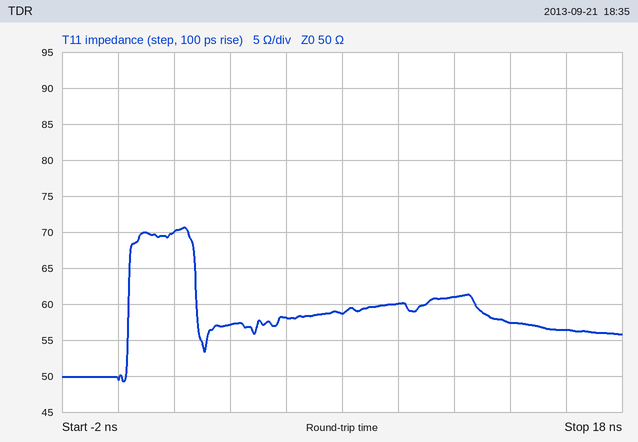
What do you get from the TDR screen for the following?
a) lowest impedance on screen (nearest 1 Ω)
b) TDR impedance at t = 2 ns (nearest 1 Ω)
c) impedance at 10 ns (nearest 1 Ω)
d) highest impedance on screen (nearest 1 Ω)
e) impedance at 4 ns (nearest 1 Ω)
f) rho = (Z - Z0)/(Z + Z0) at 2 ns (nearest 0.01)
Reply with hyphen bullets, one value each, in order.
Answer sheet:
- 49 Ω
- 70 Ω
- 60 Ω
- 71 Ω
- 57 Ω
- +0.17
